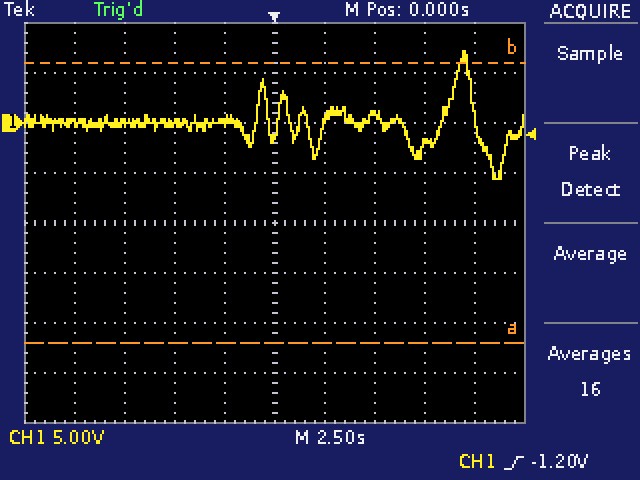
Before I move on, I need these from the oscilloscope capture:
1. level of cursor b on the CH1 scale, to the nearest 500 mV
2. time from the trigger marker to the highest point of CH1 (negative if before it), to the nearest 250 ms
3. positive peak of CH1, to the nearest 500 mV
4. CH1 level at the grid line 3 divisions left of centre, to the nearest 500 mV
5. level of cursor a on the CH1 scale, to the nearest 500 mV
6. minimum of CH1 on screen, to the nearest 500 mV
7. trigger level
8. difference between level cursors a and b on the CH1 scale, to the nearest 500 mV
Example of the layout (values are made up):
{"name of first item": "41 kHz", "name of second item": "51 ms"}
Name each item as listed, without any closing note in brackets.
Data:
{"level of cursor b on the CH1 scale, to the nearest 500 mV": "6.0 V", "time from the trigger marker to the highest point of CH1 (negative if before it), to the nearest 250 ms": "+9.50 s", "positive peak of CH1, to the nearest 500 mV": "7.0 V", "CH1 level at the grid line 3 divisions left of centre, to the nearest 500 mV": "0.0 V", "level of cursor a on the CH1 scale, to the nearest 500 mV": "-22.0 V", "minimum of CH1 on screen, to the nearest 500 mV": "-5.5 V", "trigger level": "-1.20 V", "difference between level cursors a and b on the CH1 scale, to the nearest 500 mV": "28.0 V"}
